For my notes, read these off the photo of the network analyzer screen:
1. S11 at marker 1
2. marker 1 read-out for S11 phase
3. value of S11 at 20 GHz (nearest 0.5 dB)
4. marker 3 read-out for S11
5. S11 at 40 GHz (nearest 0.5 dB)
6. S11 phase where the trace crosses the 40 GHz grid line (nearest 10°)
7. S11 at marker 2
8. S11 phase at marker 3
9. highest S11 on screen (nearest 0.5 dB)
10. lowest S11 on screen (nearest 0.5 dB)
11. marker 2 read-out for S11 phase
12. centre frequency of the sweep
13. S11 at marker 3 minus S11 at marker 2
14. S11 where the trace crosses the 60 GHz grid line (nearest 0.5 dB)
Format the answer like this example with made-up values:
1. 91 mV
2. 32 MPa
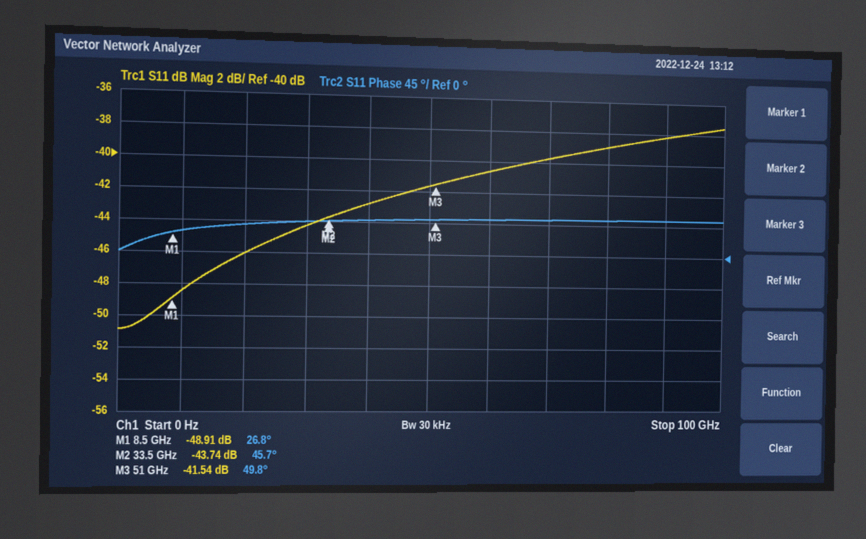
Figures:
1. -48.91 dB
2. 26.8°
3. -46.0 dB
4. -41.54 dB
5. -43.0 dB
6. 50°
7. -43.74 dB
8. 49.8°
9. -37.5 dB
10. -51.0 dB
11. 45.7°
12. 50 GHz
13. 2.20 dB
14. -40.5 dB
